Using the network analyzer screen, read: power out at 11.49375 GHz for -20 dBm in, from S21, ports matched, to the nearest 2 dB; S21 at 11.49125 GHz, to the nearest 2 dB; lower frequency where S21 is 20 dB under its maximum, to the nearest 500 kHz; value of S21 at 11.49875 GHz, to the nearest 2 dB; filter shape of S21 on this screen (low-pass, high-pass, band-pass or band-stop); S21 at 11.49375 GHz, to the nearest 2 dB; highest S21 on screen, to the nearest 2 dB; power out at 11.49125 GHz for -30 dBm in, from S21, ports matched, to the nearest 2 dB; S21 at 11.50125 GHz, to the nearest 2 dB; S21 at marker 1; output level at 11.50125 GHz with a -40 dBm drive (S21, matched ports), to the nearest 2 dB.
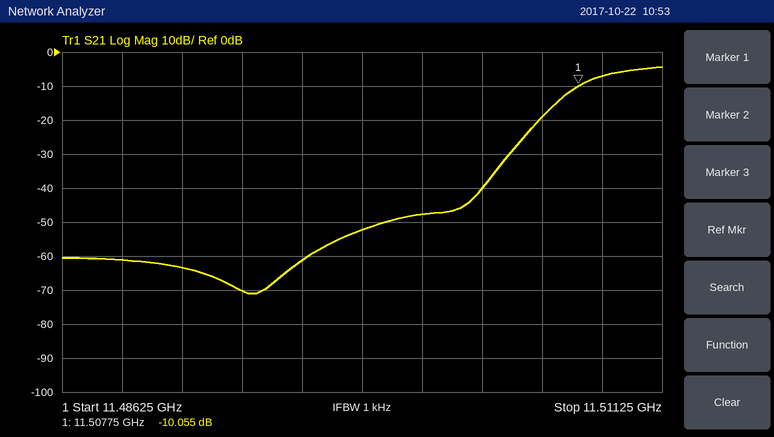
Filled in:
-90 dBm
-64 dB
11.5055 GHz
-52 dB
high-pass
-70 dB
-4 dB
-94 dBm
-48 dB
-10.055 dB
-88 dBm
